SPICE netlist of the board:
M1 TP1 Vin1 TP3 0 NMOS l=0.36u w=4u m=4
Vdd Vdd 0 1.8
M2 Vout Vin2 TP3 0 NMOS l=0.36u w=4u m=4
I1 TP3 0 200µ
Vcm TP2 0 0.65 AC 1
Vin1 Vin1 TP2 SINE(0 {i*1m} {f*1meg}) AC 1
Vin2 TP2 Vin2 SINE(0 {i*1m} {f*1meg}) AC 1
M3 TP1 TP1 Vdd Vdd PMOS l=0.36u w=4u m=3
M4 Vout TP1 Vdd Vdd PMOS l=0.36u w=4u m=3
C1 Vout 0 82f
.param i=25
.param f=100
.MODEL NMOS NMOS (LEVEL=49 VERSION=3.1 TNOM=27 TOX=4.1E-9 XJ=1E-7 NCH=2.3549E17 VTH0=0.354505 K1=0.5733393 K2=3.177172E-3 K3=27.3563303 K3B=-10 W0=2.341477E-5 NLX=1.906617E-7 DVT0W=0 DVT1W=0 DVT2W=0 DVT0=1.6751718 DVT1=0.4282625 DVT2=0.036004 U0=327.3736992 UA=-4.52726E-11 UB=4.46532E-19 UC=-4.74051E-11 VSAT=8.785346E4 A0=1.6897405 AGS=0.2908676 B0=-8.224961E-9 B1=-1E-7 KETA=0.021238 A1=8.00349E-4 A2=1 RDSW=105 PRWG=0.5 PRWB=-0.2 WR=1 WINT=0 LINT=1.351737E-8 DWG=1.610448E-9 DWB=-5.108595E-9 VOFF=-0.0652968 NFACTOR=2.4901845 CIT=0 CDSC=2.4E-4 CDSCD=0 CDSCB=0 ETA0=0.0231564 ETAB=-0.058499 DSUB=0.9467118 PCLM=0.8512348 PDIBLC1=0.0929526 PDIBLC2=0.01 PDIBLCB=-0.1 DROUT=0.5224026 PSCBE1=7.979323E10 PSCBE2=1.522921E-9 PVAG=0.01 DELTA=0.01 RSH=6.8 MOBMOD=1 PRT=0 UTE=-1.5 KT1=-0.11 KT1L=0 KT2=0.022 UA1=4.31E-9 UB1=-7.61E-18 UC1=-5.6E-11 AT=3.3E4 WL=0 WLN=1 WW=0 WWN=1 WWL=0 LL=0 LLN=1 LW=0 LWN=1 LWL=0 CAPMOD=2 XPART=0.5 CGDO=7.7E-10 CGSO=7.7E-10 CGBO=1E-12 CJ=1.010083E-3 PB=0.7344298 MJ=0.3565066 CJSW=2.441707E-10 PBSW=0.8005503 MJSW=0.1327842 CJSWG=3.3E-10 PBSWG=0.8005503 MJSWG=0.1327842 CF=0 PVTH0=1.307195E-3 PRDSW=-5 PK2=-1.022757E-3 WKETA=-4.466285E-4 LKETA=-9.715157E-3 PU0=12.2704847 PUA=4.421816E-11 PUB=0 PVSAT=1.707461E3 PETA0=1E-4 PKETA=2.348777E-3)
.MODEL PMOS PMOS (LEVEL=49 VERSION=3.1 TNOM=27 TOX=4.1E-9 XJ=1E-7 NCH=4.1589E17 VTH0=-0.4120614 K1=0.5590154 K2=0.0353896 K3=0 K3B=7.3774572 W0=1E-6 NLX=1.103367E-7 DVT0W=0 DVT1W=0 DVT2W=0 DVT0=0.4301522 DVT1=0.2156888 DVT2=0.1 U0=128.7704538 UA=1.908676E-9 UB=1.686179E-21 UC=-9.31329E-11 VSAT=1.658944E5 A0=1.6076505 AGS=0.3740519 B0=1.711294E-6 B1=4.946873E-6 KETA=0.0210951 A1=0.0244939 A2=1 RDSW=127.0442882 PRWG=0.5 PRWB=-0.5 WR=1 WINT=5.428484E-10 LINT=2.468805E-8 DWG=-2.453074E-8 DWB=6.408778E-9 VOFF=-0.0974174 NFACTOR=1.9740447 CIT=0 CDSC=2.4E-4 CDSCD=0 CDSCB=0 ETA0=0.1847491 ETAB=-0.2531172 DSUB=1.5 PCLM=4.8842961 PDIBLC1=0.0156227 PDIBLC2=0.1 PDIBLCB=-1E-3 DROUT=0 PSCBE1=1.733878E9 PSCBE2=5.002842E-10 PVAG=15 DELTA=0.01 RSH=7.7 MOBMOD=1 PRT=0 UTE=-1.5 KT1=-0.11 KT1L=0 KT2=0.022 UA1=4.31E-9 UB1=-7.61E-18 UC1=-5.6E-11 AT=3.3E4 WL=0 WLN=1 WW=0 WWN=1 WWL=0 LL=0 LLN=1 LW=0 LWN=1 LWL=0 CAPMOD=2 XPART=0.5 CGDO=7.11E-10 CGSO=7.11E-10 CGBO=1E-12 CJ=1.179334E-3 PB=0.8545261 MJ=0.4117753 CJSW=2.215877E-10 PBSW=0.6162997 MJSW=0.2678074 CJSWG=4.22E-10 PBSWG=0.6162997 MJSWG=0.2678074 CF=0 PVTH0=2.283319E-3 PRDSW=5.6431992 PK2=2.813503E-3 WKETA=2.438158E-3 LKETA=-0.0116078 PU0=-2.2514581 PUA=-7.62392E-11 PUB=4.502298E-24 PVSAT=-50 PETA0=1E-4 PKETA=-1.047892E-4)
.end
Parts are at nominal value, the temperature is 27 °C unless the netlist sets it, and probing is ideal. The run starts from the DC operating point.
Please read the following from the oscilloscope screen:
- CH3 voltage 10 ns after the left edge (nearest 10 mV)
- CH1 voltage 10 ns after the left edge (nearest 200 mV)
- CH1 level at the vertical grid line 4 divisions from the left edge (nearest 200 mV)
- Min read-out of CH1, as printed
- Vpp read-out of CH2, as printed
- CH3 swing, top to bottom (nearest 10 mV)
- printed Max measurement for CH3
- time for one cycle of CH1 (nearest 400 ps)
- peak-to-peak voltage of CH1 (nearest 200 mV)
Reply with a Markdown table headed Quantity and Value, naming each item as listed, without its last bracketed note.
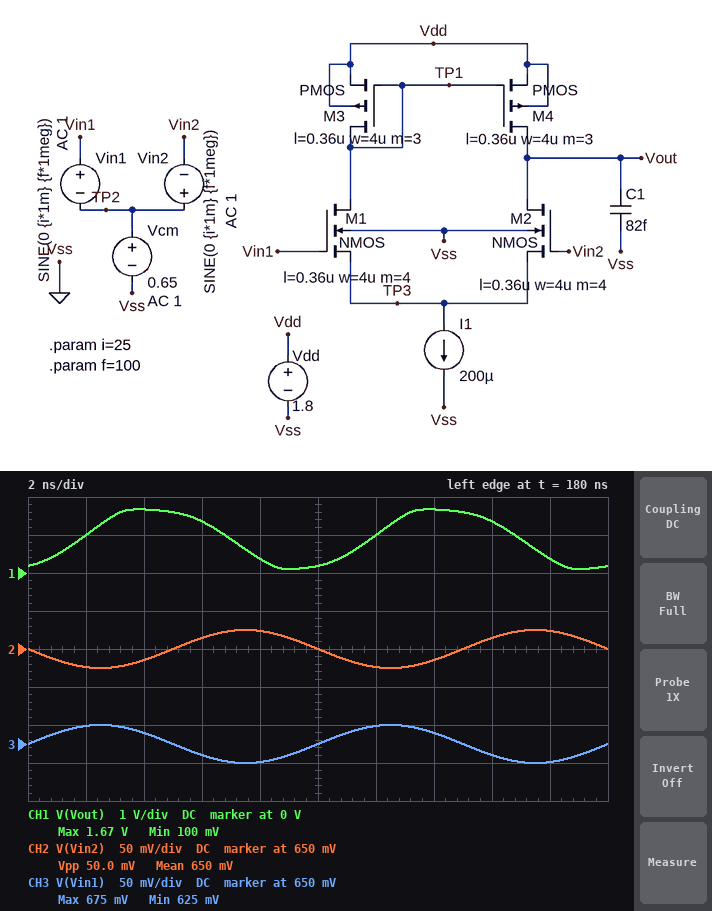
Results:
| Quantity | Value |
|---|---|
| CH3 voltage 10 ns after the left edge | 650 mV |
| CH1 voltage 10 ns after the left edge | 200 mV |
| CH1 level at the vertical grid line 4 divisions from the left edge | 400 mV |
| Min read-out of CH1, as printed | 100 mV |
| Vpp read-out of CH2, as printed | 50.0 mV |
| CH3 swing, top to bottom | 50 mV |
| printed Max measurement for CH3 | 675 mV |
| time for one cycle of CH1 | 10.0 ns |
| peak-to-peak voltage of CH1 | 1.6 V |
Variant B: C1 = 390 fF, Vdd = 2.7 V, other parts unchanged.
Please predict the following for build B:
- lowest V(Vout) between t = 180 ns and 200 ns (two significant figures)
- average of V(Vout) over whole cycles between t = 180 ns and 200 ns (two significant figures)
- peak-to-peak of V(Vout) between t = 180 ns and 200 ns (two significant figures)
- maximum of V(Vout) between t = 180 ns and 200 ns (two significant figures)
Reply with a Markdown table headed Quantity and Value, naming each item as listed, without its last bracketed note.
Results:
| Quantity | Value |
|---|---|
| lowest V(Vout) between t = 180 ns and 200 ns | 1.7 V |
| average of V(Vout) over whole cycles between t = 180 ns and 200 ns | 1.9 V |
| peak-to-peak of V(Vout) between t = 180 ns and 200 ns | 530 mV |
| maximum of V(Vout) between t = 180 ns and 200 ns | 2.2 V |
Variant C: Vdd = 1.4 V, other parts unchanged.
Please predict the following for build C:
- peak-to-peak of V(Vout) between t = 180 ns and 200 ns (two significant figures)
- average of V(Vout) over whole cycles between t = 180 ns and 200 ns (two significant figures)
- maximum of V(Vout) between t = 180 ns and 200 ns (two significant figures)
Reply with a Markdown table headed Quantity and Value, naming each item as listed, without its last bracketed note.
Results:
| Quantity | Value |
|---|---|
| peak-to-peak of V(Vout) between t = 180 ns and 200 ns | 1.2 V |
| average of V(Vout) over whole cycles between t = 180 ns and 200 ns | 680 mV |
| maximum of V(Vout) between t = 180 ns and 200 ns | 1.3 V |
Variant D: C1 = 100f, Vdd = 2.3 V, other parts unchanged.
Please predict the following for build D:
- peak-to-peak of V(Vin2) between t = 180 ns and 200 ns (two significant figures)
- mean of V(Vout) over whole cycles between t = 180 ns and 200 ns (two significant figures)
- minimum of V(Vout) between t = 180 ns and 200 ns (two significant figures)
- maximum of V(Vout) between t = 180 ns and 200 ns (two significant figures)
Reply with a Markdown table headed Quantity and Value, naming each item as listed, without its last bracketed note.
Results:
| Quantity | Value |
|---|---|
| peak-to-peak of V(Vin2) between t = 180 ns and 200 ns | 50 mV |
| mean of V(Vout) over whole cycles between t = 180 ns and 200 ns | 1.4 V |
| minimum of V(Vout) between t = 180 ns and 200 ns | 600 mV |
| maximum of V(Vout) between t = 180 ns and 200 ns | 2.1 V |
